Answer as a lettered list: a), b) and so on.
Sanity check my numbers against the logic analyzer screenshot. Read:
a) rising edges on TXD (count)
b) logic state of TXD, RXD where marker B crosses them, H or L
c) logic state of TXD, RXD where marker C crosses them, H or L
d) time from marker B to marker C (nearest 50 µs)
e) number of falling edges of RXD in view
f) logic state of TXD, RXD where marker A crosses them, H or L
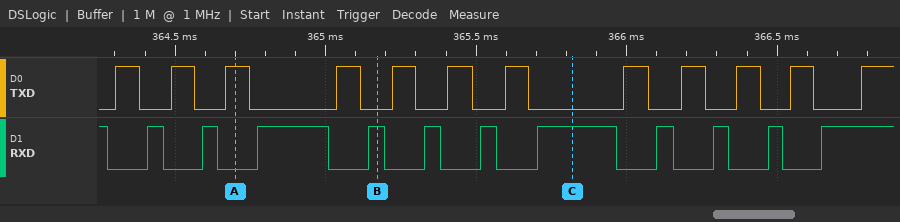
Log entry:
a) 12
b) TXD=L, RXD=H
c) TXD=L, RXD=H
d) 650 µs
e) 11
f) TXD=H, RXD=L
